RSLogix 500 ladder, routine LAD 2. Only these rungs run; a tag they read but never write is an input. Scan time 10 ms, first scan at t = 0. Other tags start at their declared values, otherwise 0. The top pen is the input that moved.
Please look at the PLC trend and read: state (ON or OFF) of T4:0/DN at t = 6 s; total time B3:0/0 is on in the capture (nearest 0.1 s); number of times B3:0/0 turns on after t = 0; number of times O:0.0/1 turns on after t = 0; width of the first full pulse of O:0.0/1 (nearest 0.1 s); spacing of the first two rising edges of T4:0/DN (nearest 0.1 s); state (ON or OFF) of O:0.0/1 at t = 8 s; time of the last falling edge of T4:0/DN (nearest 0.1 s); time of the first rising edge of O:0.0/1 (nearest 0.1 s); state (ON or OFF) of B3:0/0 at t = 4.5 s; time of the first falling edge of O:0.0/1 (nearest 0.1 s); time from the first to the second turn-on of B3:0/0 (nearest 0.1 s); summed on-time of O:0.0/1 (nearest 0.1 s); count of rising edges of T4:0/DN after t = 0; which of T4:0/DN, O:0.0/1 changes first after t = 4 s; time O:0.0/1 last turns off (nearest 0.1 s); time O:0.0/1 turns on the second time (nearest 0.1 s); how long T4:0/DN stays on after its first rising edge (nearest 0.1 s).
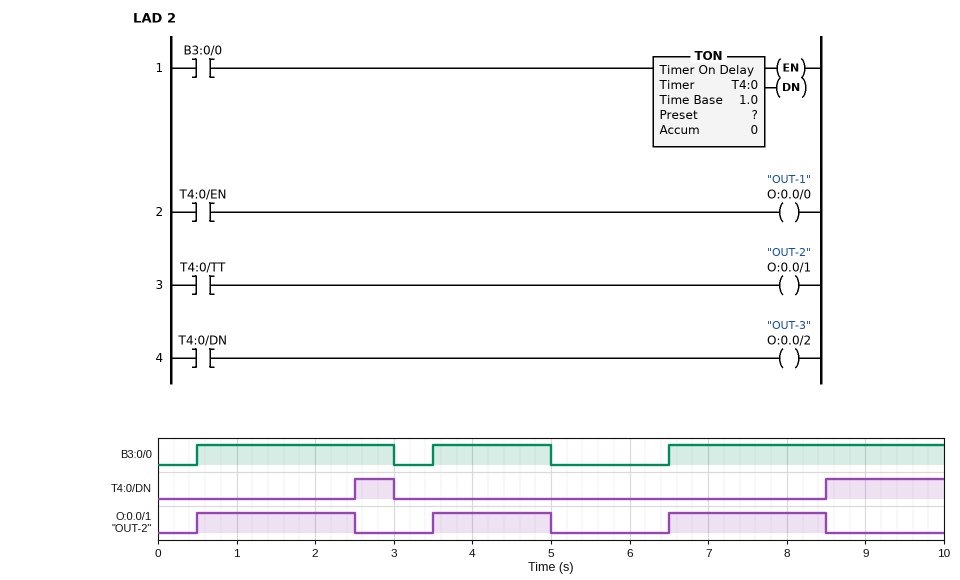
OFF
7.5 s
3
3
2.0 s
6.0 s
ON
3.0 s
0.5 s
ON
2.5 s
3.0 s
5.5 s
2
O:0.0/1
8.5 s
3.5 s
0.5 s
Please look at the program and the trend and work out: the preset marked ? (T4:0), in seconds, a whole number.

2 s
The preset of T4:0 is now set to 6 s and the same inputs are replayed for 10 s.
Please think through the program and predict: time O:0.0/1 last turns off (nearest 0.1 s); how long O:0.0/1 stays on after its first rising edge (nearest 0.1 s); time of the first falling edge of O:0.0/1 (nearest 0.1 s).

5.0 s
2.5 s
3.0 s
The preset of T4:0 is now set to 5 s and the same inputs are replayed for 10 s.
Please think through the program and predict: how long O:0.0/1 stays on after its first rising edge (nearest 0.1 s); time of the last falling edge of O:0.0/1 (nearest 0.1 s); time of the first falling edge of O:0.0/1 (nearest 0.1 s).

2.5 s
5.0 s
3.0 s
